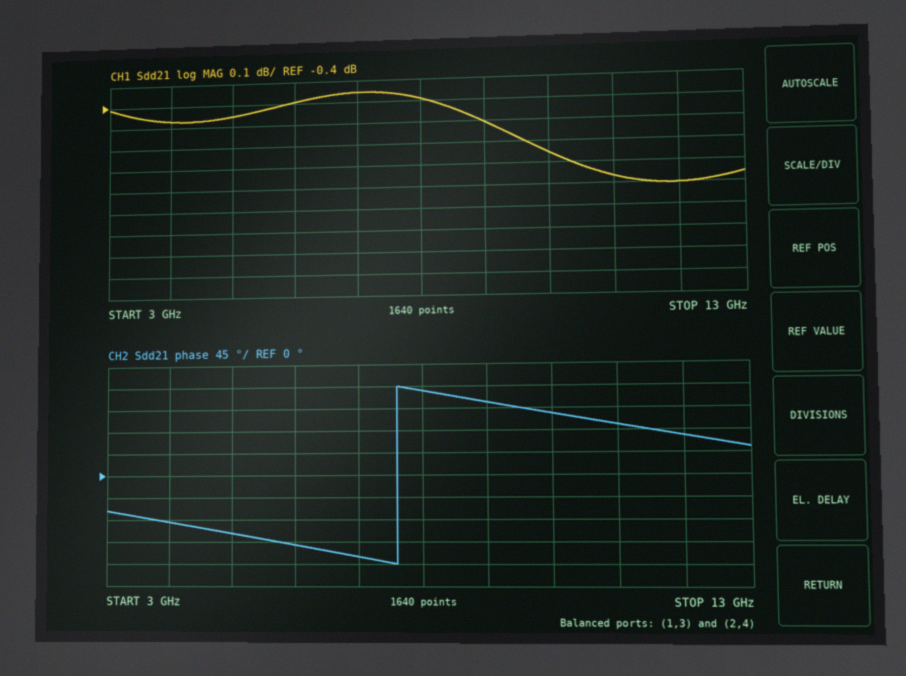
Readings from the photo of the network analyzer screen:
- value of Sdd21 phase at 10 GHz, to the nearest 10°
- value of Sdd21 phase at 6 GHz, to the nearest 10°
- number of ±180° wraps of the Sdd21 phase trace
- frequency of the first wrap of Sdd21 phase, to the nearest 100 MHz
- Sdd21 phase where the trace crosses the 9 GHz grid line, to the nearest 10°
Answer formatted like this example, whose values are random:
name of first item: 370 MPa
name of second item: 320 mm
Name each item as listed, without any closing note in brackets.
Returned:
value of Sdd21 phase at 10 GHz, to the nearest 10°: 120°
value of Sdd21 phase at 6 GHz, to the nearest 10°: -140°
number of ±180° wraps of the Sdd21 phase trace: 1
frequency of the first wrap of Sdd21 phase, to the nearest 100 MHz: 7.6 GHz
Sdd21 phase where the trace crosses the 9 GHz grid line, to the nearest 10°: 150°
